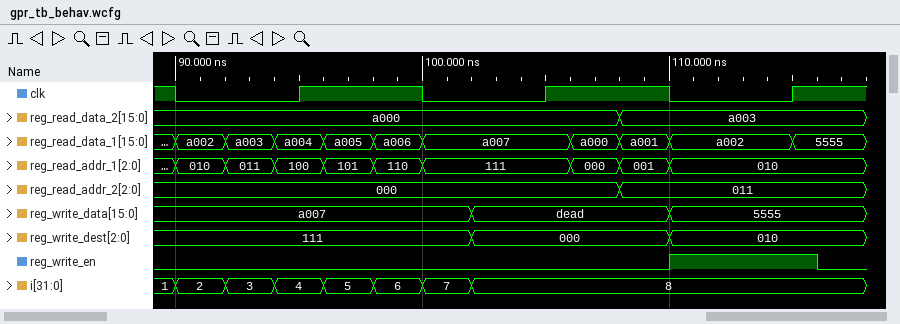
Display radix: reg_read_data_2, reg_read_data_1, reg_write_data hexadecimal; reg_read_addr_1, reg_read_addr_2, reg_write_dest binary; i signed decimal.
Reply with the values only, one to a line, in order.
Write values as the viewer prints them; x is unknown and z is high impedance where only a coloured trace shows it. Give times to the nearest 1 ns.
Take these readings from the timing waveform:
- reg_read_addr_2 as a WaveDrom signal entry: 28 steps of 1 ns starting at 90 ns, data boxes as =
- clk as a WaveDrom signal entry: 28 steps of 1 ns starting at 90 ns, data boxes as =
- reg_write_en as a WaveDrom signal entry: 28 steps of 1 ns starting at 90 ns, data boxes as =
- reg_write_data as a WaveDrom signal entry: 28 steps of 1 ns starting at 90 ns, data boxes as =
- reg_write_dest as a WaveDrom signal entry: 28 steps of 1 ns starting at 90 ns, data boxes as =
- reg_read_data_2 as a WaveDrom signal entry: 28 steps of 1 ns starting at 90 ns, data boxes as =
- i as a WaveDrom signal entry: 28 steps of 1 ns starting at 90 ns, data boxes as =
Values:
{name: 'reg_read_addr_2', wave: '=.................=.........', data: '000 011'}
{name: 'clk', wave: '0....1....0....1....0....1..'}
{name: 'reg_write_en', wave: '0...................1.....0.'}
{name: 'reg_write_data', wave: '=...........=.......=.......', data: 'a007 dead 5555'}
{name: 'reg_write_dest', wave: '=...........=.......=.......', data: '111 000 010'}
{name: 'reg_read_data_2', wave: '=.................=.........', data: 'a000 a003'}
{name: 'i', wave: '=.=.=.=.=.=.=...............', data: '2 3 4 5 6 7 8'}
